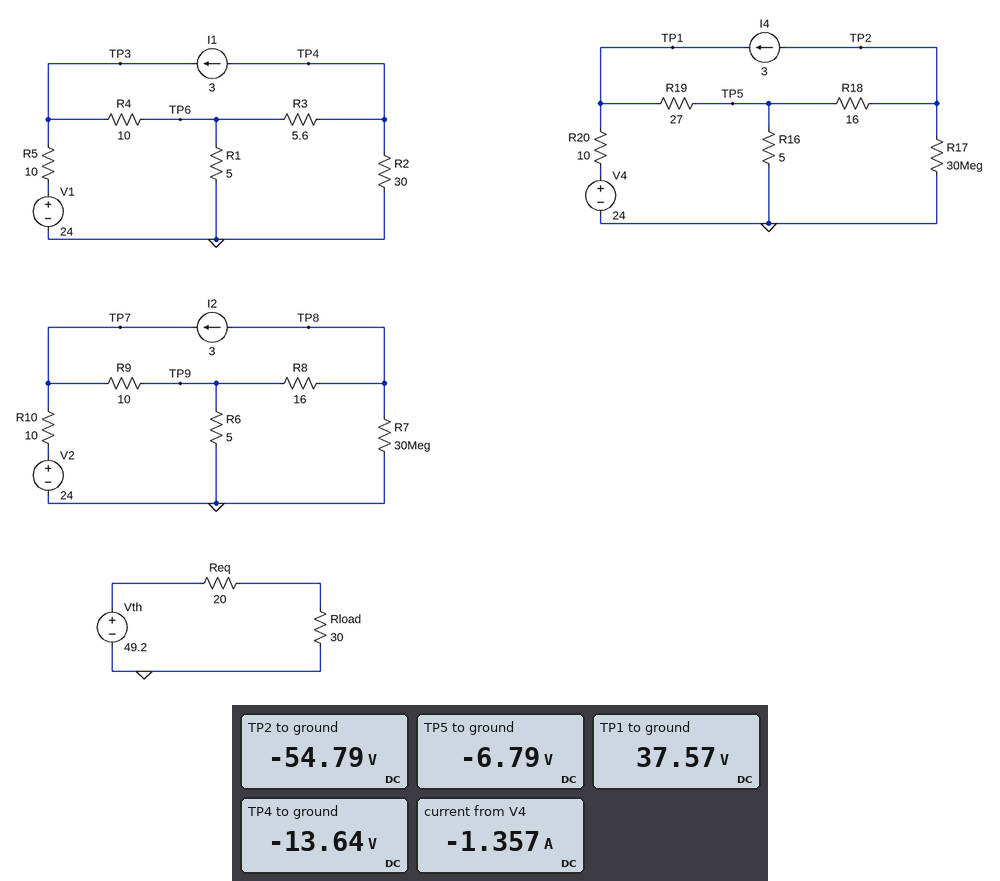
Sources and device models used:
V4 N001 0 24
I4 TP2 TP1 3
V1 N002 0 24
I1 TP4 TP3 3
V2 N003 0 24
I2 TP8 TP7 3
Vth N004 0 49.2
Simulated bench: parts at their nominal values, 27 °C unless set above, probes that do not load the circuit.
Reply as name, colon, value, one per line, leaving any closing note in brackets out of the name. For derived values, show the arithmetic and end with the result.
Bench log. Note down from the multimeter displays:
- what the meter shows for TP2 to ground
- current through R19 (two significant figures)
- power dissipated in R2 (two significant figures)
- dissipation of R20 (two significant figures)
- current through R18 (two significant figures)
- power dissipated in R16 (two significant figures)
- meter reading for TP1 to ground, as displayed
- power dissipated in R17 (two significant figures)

what the meter shows for TP2 to ground: -54.79 V
current through R19: (37.57 V - (-6.79 V)) / 27 Ω = 1.6 A
power dissipated in R2: (0 V - (-13.64 V))^2 / 30 Ω = 6.2 W
dissipation of R20: (37.57 V - 24 V)^2 / 10 Ω = 18 W
current through R18: (-6.79 V - (-54.79 V)) / 16 Ω = 3.0 A
power dissipated in R16: (0 V - (-6.79 V))^2 / 5 Ω = 9.2 W
meter reading for TP1 to ground, as displayed: 37.57 V
power dissipated in R17: (0 V - (-54.79 V))^2 / 30 MΩ = 100 µW
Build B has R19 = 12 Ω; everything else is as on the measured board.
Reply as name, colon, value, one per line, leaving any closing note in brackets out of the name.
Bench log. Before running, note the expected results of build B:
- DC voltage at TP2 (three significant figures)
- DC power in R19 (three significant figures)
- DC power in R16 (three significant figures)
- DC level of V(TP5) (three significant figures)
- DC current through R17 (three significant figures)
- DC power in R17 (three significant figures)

DC voltage at TP2: -50.2 V
DC power in R19: 78.4 W
DC power in R16: 988 mW
DC level of V(TP5): -2.22 V
DC current through R17: 1.67 µA
DC power in R17: 84.1 µW
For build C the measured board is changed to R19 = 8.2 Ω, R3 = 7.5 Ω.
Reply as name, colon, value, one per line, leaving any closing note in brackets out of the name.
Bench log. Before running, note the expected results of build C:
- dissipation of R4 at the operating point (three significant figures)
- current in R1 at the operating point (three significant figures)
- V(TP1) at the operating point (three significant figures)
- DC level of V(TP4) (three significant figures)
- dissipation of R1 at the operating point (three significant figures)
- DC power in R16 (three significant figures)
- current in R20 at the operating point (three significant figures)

dissipation of R4 at the operating point: 70.0 W
current in R1 at the operating point: 217 mA
V(TP1) at the operating point: 24.3 V
DC level of V(TP4): -17.1 V
dissipation of R1 at the operating point: 235 mW
DC power in R16: 3.34 mW
current in R20 at the operating point: 25.9 mA
